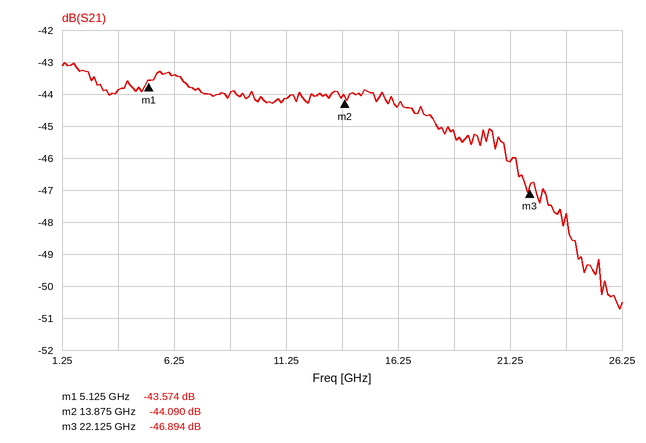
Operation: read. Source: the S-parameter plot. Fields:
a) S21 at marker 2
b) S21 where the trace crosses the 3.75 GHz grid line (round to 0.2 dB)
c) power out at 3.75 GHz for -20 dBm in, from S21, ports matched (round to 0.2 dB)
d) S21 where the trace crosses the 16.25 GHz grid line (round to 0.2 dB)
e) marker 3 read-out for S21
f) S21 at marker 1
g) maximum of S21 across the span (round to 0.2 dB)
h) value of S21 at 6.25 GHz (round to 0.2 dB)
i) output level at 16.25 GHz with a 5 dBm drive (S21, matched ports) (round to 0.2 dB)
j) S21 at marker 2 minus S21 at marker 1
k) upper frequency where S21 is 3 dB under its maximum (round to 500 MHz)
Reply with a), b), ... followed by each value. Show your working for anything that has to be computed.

a) -44.090 dB
b) -43.8 dB
c) -20 dBm + (-43.8 dB) = -63.8 dBm
d) -44.4 dB
e) -46.894 dB
f) -43.574 dB
g) -43.0 dB
h) -43.4 dB
i) 5 dBm + (-44.4 dB) = -39.4 dBm
j) -44.09 − (-43.574) = -0.516 dB
k) 21.0 GHz
